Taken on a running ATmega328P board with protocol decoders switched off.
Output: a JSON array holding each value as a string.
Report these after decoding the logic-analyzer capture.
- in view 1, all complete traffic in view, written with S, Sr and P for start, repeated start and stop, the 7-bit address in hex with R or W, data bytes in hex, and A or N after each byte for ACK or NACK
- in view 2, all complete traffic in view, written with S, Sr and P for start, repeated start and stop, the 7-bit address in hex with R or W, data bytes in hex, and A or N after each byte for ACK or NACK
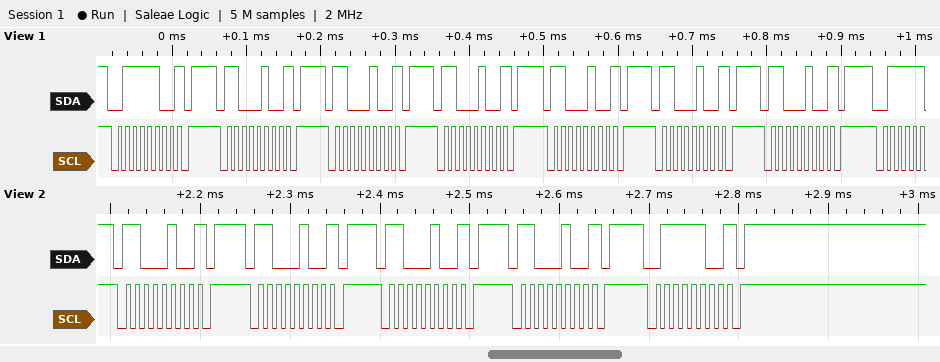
["S 3EW N P S 62W N P S 62W N P S 62W N P S 62W N P S 62W N P S 62W N P", "S 62W N P S 62W N P S 62W N P S 62W N P S 3EW N P"]
